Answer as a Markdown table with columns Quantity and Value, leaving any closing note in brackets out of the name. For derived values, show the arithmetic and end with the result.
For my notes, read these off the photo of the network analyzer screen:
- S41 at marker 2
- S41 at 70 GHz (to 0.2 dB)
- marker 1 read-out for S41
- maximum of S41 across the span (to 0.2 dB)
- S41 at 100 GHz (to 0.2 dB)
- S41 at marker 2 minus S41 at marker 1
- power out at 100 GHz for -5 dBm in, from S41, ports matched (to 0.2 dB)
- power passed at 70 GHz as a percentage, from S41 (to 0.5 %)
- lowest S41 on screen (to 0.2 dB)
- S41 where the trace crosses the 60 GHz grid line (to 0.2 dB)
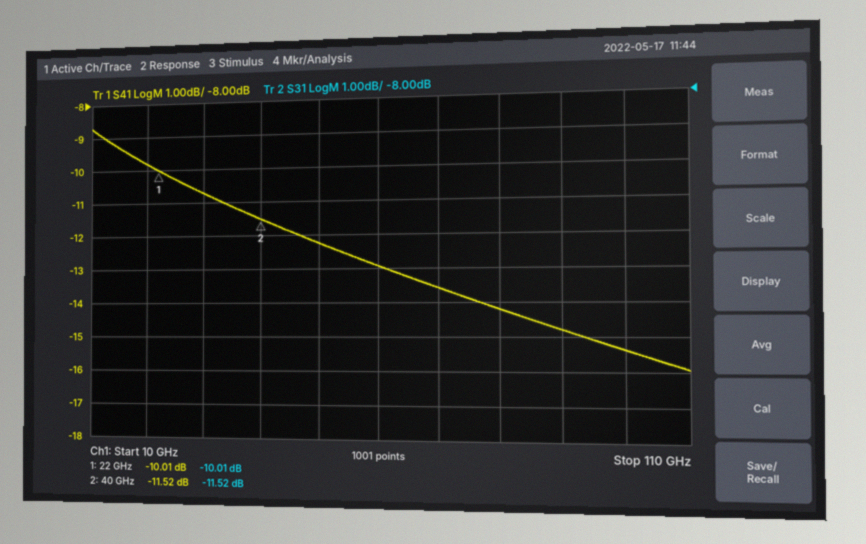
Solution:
| Quantity | Value |
|---|---|
| S41 at marker 2 | -11.52 dB |
| S41 at 70 GHz | -13.6 dB |
| marker 1 read-out for S41 | -10.01 dB |
| maximum of S41 across the span | -8.8 dB |
| S41 at 100 GHz | -15.4 dB |
| S41 at marker 2 minus S41 at marker 1 | -11.52 − (-10.01) = -1.51 dB |
| power out at 100 GHz for -5 dBm in, from S41, ports matched | -5 dBm + (-15.4 dB) = -20.4 dBm |
| power passed at 70 GHz as a percentage, from S41 | 10^(-13.6/10) ≈ 4.37 %, so 4.5 % to the nearest 0.5 % |
| lowest S41 on screen | -16.0 dB |
| S41 where the trace crosses the 60 GHz grid line | -13.0 dB |
